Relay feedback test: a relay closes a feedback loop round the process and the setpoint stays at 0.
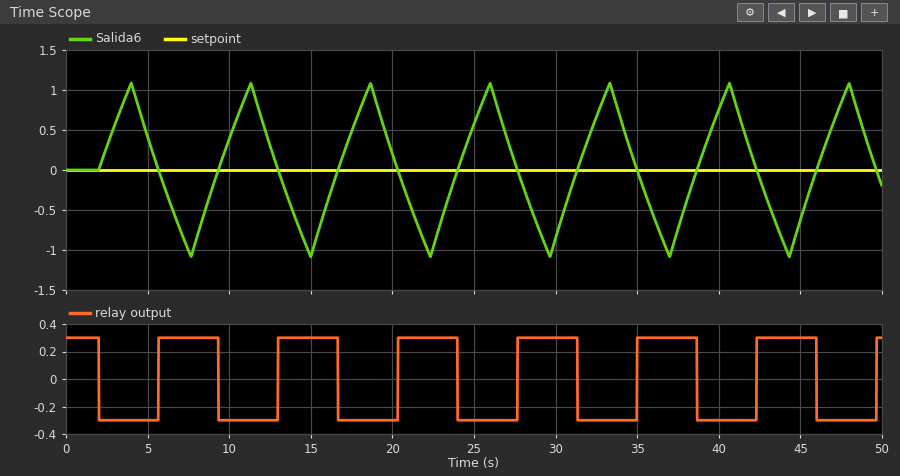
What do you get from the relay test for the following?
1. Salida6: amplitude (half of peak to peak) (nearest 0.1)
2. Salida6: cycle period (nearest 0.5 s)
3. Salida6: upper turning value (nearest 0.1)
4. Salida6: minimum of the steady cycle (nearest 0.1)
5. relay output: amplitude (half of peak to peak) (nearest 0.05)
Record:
1.1
7.5 s
1.1
-1.1
0.30
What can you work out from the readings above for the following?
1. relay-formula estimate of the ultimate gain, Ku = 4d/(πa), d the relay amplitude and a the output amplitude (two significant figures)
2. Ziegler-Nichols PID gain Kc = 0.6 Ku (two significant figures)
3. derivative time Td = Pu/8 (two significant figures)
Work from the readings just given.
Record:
0.35
0.21
0.94 s
